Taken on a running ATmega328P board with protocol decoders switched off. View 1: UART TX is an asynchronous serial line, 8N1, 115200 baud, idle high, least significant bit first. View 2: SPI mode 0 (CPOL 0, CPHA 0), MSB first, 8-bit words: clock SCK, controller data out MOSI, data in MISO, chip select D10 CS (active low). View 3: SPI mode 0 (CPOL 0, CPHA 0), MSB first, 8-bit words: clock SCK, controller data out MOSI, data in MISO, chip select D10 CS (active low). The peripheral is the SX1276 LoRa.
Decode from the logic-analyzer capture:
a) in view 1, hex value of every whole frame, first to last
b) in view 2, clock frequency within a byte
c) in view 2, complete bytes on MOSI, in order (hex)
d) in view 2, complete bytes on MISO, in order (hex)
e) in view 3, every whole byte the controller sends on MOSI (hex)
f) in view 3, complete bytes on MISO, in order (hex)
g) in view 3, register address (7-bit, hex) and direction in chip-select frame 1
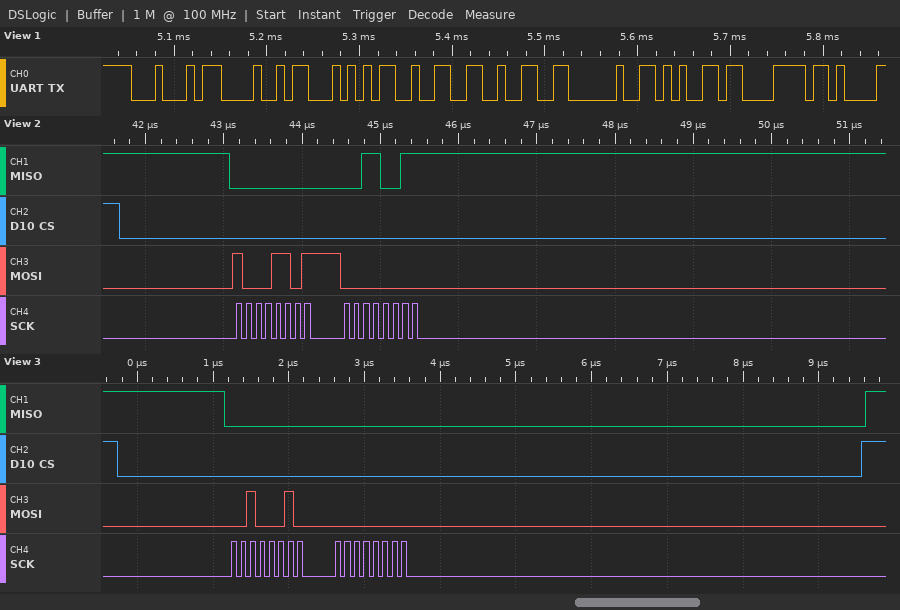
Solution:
44 48 54 32 32 20 65 78
8 MHz
0x8D 0x00
0x00 0x33
22 00
00 00
0x22 read
